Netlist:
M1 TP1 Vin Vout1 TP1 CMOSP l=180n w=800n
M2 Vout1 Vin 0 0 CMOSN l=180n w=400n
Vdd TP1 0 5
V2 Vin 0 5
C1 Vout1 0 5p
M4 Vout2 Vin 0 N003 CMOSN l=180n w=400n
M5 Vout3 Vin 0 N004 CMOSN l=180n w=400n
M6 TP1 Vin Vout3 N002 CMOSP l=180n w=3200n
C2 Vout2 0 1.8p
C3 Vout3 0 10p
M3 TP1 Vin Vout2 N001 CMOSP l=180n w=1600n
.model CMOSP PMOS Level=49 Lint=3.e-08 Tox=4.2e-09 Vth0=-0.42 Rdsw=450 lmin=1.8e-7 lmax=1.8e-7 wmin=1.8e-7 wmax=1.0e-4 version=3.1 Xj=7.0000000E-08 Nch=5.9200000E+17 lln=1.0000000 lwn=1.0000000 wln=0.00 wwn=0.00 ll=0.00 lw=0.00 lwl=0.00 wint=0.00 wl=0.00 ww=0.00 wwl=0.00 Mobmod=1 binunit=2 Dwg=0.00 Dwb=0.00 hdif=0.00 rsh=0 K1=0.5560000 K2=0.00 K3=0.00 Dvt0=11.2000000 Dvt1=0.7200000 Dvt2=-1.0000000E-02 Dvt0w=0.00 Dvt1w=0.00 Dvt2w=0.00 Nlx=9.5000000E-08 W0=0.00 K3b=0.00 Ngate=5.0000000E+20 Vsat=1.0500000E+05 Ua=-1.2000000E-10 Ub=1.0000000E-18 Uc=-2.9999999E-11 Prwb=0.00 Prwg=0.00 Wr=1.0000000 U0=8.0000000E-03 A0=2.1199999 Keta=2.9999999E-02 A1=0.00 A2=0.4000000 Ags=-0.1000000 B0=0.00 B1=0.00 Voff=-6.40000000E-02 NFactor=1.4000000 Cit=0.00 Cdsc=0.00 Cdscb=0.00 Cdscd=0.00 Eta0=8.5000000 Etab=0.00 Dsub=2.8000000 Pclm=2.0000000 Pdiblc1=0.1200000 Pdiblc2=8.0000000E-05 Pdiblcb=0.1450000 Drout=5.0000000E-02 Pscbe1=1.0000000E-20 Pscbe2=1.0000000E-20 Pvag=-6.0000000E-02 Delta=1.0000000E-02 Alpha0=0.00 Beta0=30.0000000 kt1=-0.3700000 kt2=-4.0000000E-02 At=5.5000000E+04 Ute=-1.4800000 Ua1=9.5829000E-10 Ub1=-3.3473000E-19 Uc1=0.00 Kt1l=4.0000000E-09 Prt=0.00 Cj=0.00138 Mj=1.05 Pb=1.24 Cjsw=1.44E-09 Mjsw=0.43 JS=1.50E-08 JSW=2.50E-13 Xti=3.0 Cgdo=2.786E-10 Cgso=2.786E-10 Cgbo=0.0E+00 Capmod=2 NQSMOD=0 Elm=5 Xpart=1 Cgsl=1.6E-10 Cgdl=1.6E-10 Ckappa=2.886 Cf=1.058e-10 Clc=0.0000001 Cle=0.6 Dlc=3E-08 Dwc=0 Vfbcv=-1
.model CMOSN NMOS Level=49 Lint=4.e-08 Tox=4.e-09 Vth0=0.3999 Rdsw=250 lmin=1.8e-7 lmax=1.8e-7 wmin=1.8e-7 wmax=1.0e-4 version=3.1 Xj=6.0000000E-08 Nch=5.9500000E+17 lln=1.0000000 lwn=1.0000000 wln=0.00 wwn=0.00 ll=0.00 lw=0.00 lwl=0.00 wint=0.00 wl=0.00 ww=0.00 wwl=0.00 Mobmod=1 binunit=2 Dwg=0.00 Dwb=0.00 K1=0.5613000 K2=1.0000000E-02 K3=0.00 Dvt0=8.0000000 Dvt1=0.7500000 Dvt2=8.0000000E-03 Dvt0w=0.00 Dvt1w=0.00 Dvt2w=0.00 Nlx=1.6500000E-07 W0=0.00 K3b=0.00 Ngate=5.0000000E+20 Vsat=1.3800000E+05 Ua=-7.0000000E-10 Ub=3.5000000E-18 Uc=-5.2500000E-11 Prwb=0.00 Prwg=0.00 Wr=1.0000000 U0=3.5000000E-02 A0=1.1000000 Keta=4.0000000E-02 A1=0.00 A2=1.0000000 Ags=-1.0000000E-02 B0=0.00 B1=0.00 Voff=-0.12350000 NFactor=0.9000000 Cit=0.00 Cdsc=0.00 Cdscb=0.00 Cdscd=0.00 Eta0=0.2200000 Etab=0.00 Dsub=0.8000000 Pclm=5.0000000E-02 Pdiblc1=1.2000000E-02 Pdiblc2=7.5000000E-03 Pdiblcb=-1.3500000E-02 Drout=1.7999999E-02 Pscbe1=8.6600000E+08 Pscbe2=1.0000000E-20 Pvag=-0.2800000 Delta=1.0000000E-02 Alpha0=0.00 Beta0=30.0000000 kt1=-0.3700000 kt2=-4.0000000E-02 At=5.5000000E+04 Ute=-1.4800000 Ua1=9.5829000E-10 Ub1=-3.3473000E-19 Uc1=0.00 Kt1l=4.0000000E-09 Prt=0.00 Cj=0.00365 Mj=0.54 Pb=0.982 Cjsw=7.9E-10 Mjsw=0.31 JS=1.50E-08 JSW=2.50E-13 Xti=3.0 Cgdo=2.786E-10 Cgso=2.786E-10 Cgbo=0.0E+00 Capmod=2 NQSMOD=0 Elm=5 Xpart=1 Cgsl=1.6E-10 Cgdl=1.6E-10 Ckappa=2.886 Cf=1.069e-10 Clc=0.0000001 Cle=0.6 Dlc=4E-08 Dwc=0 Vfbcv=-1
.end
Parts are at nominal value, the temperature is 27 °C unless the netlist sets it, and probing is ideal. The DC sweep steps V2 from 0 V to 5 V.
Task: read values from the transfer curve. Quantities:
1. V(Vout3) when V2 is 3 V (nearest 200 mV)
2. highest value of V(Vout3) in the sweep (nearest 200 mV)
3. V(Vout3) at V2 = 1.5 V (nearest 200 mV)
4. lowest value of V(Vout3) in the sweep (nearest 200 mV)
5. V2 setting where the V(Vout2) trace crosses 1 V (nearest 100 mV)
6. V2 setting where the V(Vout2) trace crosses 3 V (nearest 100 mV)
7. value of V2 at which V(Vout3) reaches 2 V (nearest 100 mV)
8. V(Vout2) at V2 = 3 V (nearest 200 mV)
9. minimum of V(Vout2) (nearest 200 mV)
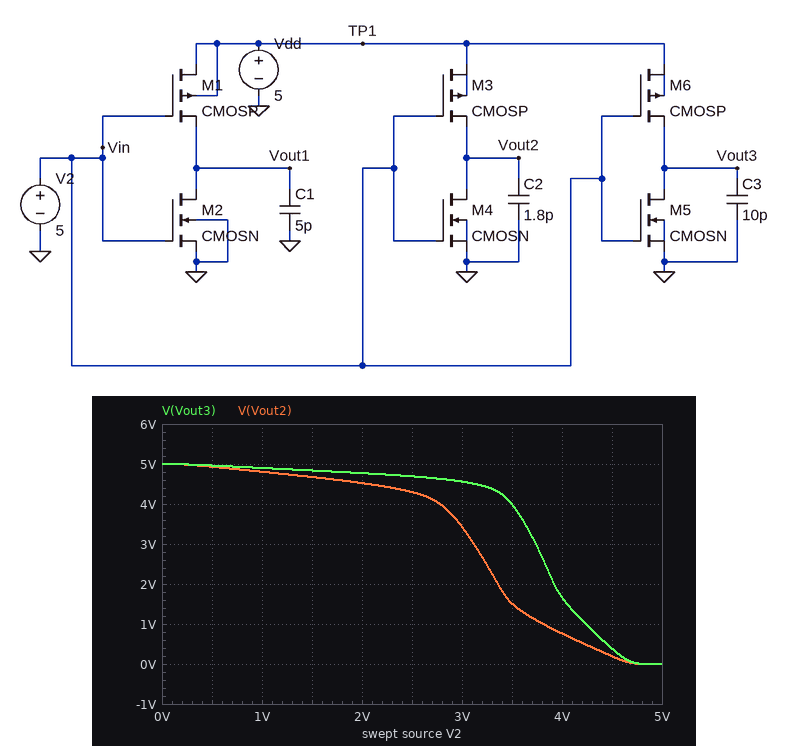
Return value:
4.6 V
5.0 V
4.8 V
0 V
3.8 V
3.1 V
3.9 V
3.4 V
0 V
